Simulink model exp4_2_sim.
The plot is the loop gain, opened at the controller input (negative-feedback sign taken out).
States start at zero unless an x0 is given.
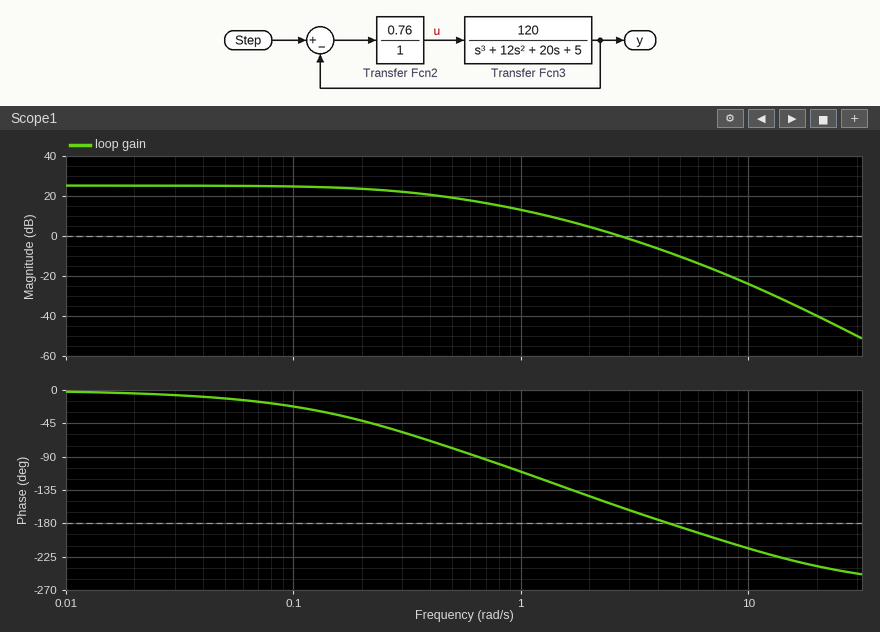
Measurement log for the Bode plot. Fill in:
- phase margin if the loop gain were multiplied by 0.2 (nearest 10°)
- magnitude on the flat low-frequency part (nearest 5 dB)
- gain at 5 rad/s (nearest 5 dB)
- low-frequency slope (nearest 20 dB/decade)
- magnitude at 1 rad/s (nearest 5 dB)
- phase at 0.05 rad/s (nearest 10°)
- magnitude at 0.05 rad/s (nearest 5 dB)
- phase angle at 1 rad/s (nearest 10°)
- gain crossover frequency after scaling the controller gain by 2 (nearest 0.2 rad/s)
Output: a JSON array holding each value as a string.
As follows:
["70°", "25 dB", "-10 dB", "0 dB/decade", "15 dB", "-10°", "25 dB", "-110°", "4.0 rad/s"]
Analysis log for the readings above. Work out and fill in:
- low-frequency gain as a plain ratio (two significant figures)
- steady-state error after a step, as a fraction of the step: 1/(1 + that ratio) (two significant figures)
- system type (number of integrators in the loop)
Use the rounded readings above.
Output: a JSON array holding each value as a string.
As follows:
["18", "0.053", "0"]
